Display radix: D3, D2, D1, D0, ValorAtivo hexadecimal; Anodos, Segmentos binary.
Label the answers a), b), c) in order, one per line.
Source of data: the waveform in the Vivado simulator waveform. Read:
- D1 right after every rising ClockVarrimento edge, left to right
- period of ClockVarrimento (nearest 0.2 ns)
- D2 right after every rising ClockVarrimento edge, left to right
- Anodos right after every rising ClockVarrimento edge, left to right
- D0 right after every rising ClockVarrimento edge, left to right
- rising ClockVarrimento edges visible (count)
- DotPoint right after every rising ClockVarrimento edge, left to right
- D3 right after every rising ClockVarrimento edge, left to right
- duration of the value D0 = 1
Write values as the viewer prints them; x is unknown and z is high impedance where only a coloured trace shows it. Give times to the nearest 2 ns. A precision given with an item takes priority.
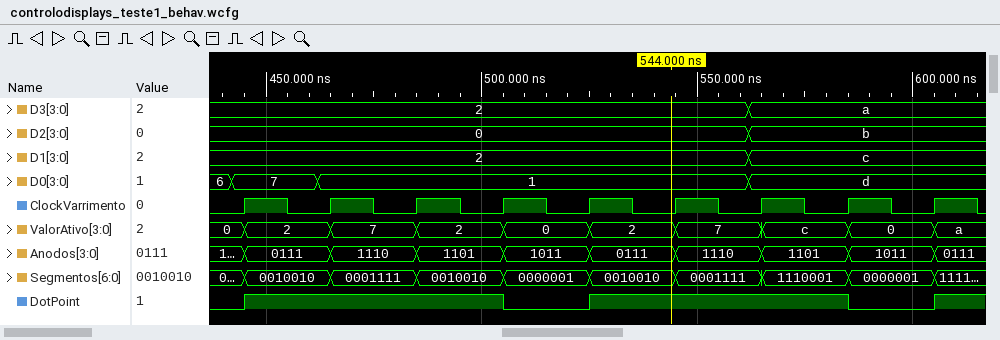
a) 2, 2, 2, 2, 2, 2, c, c, c
b) 20 ns
c) 0, 0, 0, 0, 0, 0, b, b, b
d) 0111, 1110, 1101, 1011, 0111, 1110, 1101, 1011, 0111
e) 7, 1, 1, 1, 1, 1, d, d, d
f) 9
g) 1 1 1 0 1 1 1 0 1
h) 2, 2, 2, 2, 2, 2, a, a, a
i) 100 ns
